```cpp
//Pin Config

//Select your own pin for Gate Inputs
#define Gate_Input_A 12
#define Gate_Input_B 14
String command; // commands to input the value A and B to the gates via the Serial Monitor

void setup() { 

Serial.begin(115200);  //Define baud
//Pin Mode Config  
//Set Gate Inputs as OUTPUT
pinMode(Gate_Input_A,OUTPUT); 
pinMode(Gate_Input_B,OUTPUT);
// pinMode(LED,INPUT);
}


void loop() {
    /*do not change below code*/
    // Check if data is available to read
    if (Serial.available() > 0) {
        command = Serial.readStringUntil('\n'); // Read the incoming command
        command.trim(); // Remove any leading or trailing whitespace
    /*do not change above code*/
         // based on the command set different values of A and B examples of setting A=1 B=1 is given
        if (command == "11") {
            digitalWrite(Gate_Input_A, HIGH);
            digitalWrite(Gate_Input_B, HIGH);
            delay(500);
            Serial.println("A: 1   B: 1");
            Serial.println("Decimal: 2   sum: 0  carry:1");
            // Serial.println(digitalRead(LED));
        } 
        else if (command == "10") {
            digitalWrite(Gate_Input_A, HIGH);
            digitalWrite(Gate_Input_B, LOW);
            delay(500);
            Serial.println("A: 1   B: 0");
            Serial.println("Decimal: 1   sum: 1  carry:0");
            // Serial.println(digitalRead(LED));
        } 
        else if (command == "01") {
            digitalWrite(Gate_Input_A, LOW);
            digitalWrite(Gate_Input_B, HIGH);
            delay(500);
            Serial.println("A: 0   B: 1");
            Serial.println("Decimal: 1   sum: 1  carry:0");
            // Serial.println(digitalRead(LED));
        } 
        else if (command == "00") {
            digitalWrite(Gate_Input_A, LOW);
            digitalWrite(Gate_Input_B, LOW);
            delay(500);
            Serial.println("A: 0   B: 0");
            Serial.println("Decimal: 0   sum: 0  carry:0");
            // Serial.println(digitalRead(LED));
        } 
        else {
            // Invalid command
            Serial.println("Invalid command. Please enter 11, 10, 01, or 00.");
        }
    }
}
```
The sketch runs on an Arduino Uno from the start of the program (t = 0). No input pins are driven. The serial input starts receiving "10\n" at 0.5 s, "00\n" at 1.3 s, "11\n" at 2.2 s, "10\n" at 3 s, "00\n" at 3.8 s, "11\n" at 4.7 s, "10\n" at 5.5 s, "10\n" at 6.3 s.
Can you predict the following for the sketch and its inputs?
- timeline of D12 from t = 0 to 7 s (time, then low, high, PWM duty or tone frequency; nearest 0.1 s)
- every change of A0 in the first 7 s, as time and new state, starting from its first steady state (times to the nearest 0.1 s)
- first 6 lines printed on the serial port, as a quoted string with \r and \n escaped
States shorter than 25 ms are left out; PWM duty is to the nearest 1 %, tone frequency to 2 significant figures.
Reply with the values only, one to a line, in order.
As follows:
0 s low; 0.5 s high; 1.3 s low; 2.2 s high; 3.8 s low; 4.7 s high
0 s low; 2.2 s high; 3 s low; 4.7 s high; 5.5 s low
"A: 1   B: 0\r\nDecimal: 1   sum: 1  carry:0\r\nA: 0   B: 0\r\nDecimal: 0   sum: 0  carry:0\r\nA: 1   B: 1\r\nDecimal: 2   sum: 0  carry:1\r\n"
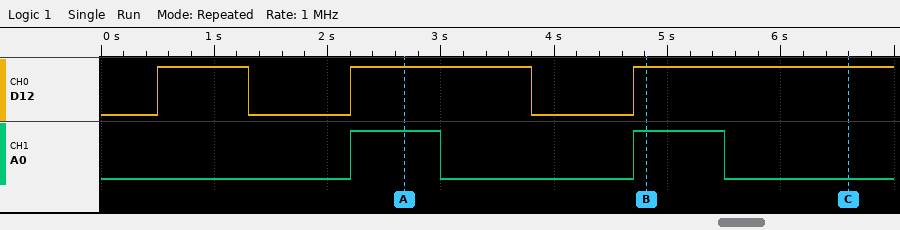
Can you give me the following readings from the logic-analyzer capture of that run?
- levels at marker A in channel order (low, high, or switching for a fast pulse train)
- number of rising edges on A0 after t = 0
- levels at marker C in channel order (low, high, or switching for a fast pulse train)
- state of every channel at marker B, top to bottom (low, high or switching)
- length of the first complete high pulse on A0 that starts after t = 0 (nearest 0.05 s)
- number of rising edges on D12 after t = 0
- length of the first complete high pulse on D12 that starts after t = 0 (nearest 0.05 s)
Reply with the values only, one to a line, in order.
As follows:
D12 high, A0 high
2
D12 high, A0 low
D12 high, A0 high
0.80 s
3
0.80 s
